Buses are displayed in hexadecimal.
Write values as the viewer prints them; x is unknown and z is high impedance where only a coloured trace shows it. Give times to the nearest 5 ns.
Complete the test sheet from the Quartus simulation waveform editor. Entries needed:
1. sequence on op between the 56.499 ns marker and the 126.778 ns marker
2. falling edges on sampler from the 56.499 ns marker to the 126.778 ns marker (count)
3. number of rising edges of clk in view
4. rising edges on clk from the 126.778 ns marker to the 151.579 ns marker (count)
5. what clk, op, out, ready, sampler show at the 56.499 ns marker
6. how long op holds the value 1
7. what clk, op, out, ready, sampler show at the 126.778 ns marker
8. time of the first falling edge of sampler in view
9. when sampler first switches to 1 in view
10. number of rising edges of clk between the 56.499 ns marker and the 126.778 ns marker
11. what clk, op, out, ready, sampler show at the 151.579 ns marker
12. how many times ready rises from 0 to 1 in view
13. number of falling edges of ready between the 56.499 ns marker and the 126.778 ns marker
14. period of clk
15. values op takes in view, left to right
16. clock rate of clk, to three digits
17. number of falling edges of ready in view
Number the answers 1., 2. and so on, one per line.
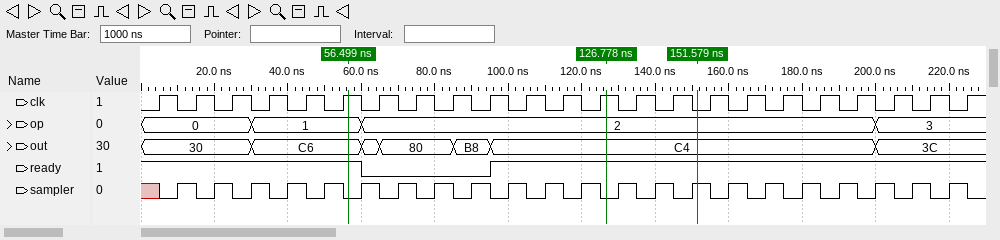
1. 1, 2
2. 7
3. 23
4. 2
5. clk=1, op=1, out=C6, ready=1, sampler=0
6. 30 ns
7. clk=1, op=2, out=C4, ready=1, sampler=0
8. 15 ns
9. 10 ns
10. 7
11. clk=0, op=2, out=C4, ready=1, sampler=1
12. 1
13. 1
14. 10 ns
15. 0, 1, 2, 3
16. 100 MHz
17. 1
